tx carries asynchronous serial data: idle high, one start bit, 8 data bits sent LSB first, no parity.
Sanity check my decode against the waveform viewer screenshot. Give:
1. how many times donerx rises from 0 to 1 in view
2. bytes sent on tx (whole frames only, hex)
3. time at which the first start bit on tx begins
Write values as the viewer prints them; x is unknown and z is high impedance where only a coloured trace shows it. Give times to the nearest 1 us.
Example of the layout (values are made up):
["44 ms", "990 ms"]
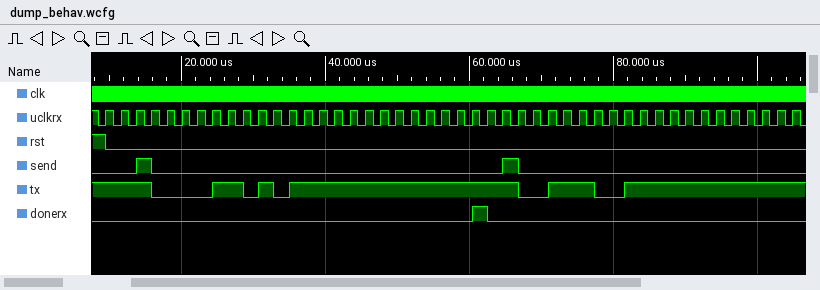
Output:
["1", "58, CE", "16 us"]
